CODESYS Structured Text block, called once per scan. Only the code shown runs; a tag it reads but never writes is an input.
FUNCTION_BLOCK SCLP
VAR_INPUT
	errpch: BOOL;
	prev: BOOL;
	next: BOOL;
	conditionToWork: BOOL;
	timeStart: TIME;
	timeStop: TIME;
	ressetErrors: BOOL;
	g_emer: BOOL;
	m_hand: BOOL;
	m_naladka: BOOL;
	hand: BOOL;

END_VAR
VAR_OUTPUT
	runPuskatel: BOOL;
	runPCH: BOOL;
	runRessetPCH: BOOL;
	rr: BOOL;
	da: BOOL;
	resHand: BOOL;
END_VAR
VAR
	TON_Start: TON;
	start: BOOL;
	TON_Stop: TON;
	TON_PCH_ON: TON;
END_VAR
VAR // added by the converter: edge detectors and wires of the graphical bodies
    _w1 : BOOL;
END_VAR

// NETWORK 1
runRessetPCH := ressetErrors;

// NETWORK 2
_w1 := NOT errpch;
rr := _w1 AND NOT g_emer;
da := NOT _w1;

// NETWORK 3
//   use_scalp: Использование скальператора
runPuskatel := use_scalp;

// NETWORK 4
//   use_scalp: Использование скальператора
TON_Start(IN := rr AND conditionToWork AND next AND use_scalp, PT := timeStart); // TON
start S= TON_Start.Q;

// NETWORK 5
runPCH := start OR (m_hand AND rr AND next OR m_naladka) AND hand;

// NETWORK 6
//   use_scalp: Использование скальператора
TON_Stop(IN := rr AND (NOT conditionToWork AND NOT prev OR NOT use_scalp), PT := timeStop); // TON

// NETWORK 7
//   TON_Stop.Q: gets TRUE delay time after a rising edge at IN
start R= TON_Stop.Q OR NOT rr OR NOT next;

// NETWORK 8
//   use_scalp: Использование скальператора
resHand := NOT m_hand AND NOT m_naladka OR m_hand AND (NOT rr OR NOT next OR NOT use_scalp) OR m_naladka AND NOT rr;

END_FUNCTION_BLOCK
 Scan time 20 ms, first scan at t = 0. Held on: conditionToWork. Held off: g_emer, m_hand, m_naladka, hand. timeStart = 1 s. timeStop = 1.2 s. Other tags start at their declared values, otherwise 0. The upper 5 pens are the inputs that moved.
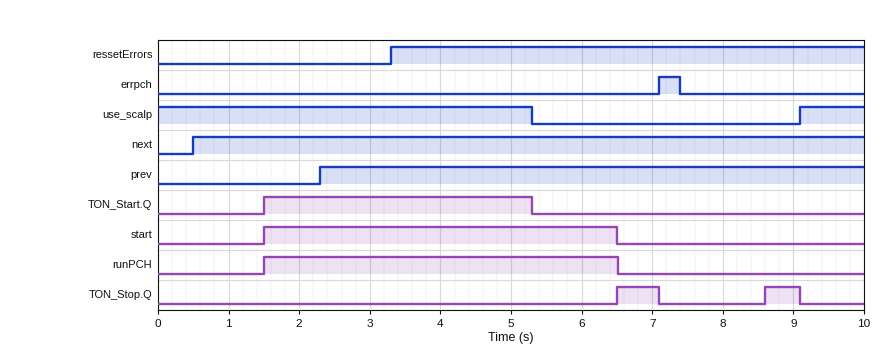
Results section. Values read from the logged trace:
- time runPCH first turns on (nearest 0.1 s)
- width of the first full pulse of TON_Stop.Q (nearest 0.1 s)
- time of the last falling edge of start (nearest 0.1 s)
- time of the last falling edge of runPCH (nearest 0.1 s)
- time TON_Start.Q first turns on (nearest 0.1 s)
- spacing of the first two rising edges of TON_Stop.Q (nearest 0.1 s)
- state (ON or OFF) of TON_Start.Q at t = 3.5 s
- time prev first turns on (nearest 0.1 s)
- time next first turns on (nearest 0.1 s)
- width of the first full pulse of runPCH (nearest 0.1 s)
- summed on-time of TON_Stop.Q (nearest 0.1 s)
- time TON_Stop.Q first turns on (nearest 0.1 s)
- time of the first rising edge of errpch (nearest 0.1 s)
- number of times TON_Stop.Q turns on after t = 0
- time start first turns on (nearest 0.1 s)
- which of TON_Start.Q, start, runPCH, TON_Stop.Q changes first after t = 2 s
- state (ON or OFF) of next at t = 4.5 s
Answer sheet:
1.5 s
0.6 s
6.5 s
6.5 s
1.5 s
2.1 s
ON
2.3 s
0.5 s
5.0 s
1.1 s
6.5 s
7.1 s
2
1.5 s
TON_Start.Q
ON
